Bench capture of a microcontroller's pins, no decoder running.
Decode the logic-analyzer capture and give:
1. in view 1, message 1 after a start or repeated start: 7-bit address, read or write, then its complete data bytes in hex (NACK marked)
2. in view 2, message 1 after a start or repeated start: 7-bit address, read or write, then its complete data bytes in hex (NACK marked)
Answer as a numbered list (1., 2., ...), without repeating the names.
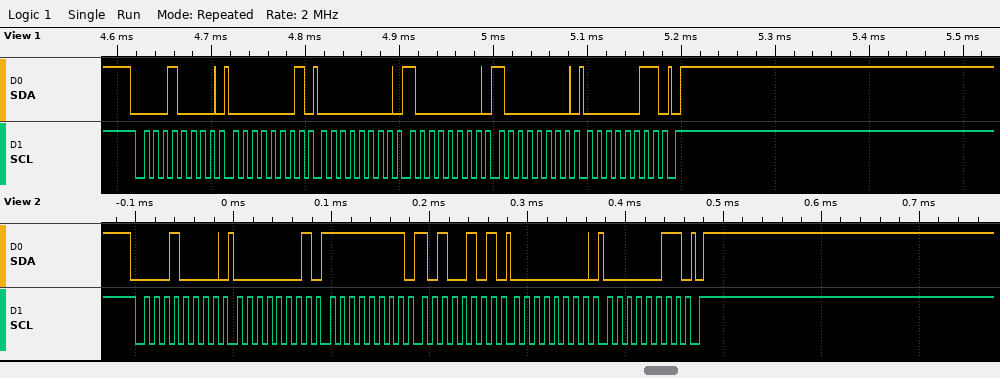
1. 0x08 write: 01 00 80 80 03
2. 0x08 write: 01 FF A5 00 03
